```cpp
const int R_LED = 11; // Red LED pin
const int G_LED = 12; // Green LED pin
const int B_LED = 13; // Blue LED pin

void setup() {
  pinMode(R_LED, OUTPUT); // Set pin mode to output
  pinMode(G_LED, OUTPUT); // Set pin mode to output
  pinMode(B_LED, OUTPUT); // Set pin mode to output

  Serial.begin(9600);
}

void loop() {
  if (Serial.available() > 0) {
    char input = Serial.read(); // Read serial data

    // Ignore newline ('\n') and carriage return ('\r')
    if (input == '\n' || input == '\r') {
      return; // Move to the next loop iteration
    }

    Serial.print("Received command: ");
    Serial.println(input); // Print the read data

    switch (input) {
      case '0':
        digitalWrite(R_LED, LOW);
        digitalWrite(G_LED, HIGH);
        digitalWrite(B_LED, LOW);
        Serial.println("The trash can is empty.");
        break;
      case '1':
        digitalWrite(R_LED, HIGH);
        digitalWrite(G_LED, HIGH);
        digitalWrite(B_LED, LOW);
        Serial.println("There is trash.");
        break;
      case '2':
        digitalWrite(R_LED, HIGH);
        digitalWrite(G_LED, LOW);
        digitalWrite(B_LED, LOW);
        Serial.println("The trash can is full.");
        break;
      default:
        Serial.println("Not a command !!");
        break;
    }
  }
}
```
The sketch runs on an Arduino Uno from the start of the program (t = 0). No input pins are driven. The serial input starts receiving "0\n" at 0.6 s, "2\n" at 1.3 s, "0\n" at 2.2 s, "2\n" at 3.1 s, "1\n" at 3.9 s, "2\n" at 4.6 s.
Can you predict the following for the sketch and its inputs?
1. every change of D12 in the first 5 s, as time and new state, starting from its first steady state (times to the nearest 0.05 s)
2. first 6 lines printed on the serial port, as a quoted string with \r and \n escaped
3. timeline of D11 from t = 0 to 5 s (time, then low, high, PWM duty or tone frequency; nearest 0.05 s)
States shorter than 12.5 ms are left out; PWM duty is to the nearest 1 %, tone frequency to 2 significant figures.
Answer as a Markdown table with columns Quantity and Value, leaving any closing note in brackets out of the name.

| Quantity | Value |
|---|---|
| every change of D12 in the first 5 s, as time and new state, starting from its first steady state | 0 s low; 0.6 s high; 1.3 s low; 2.2 s high; 3.1 s low; 3.9 s high; 4.6 s low |
| first 6 lines printed on the serial port, as a quoted string with \r and \n escaped | "Received command: 0\r\nThe trash can is empty.\r\nReceived command: 2\r\nThe trash can is full.\r\nReceived command: 0\r\nThe trash can is empty.\r\n" |
| timeline of D11 from t = 0 to 5 s | 0 s low; 1.3 s high; 2.2 s low; 3.1 s high |
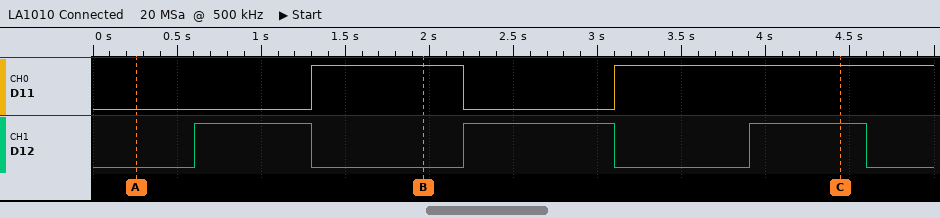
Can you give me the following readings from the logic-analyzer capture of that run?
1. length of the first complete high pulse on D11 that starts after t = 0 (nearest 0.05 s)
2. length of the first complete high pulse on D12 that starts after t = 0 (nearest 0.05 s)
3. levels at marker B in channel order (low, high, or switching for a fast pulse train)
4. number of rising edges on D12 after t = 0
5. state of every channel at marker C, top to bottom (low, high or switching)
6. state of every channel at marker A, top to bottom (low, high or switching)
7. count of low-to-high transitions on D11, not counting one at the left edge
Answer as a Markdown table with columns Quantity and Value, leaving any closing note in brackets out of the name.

| Quantity | Value |
|---|---|
| length of the first complete high pulse on D11 that starts after t = 0 | 0.90 s |
| length of the first complete high pulse on D12 that starts after t = 0 | 0.70 s |
| levels at marker B in channel order | D11 high, D12 low |
| number of rising edges on D12 after t = 0 | 3 |
| state of every channel at marker C, top to bottom | D11 high, D12 high |
| state of every channel at marker A, top to bottom | D11 low, D12 low |
| count of low-to-high transitions on D11, not counting one at the left edge | 2 |
